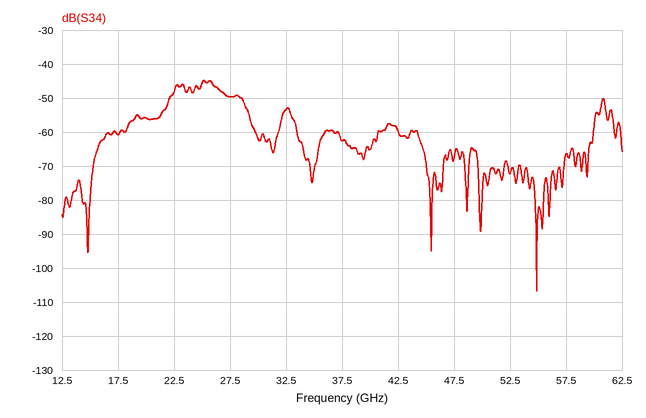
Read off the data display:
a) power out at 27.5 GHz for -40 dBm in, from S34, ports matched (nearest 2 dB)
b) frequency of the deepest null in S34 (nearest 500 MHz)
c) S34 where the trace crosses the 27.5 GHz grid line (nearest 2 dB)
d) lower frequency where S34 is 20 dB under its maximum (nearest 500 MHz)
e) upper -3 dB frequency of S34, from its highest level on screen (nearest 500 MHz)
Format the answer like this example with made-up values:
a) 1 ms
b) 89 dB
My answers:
a) -90 dBm
b) 55.0 GHz
c) -50 dB
d) 15.5 GHz
e) 26.5 GHz
